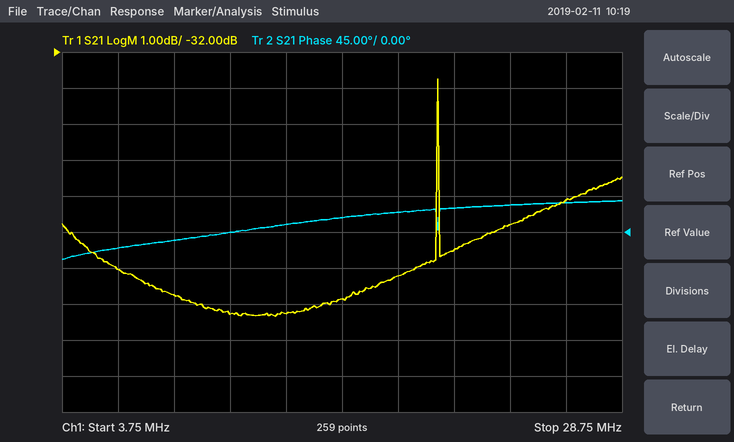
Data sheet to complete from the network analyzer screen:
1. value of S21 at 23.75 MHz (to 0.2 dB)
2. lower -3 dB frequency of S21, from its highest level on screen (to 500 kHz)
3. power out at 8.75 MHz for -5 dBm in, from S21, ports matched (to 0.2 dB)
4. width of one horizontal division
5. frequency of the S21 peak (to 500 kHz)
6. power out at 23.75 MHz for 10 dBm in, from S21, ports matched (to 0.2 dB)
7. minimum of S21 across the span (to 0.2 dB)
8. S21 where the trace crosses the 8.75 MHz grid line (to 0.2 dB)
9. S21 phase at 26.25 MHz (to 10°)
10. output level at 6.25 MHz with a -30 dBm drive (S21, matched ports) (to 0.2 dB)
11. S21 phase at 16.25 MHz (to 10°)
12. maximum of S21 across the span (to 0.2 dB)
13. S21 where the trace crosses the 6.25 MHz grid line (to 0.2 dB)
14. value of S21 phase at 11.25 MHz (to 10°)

-36.8 dB
20.5 MHz
-43.8 dBm
2.5 MHz
20.5 MHz
-26.8 dBm
-39.4 dB
-38.8 dB
40°
-68.0 dBm
20°
-32.8 dB
-38.0 dB
0°
